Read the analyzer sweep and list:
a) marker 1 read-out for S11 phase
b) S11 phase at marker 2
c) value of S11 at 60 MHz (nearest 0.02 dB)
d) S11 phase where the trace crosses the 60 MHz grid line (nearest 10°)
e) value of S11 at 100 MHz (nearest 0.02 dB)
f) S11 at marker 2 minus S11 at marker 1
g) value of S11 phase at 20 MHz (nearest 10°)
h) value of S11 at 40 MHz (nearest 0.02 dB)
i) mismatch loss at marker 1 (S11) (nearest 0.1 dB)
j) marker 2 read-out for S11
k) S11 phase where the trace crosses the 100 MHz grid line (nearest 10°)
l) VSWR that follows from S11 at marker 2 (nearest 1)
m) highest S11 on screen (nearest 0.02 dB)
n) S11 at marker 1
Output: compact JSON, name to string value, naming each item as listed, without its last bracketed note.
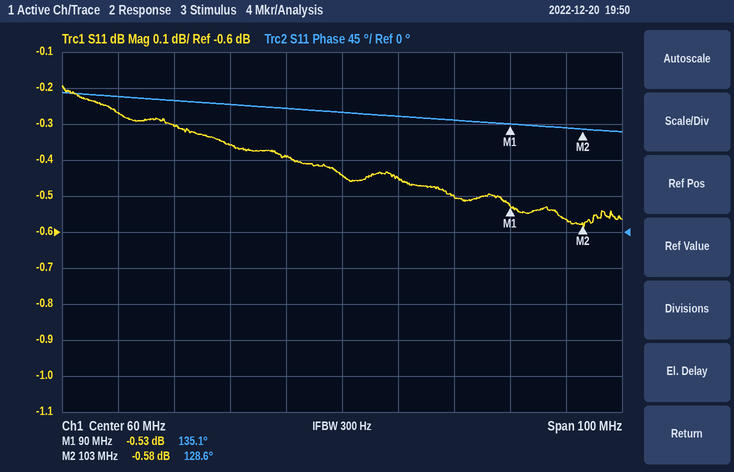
{"marker 1 read-out for S11 phase": "135.1°", "S11 phase at marker 2": "128.6°", "value of S11 at 60 MHz": "-0.44 dB", "S11 phase where the trace crosses the 60 MHz grid line": "150°", "value of S11 at 100 MHz": "-0.56 dB", "S11 at marker 2 minus S11 at marker 1": "-0.05 dB", "value of S11 phase at 20 MHz": "170°", "value of S11 at 40 MHz": "-0.36 dB", "mismatch loss at marker 1 (S11)": "9.4 dB", "marker 2 read-out for S11": "-0.58 dB", "S11 phase where the trace crosses the 100 MHz grid line": "130°", "VSWR that follows from S11 at marker 2": "30", "highest S11 on screen": "-0.20 dB", "S11 at marker 1": "-0.53 dB"}
